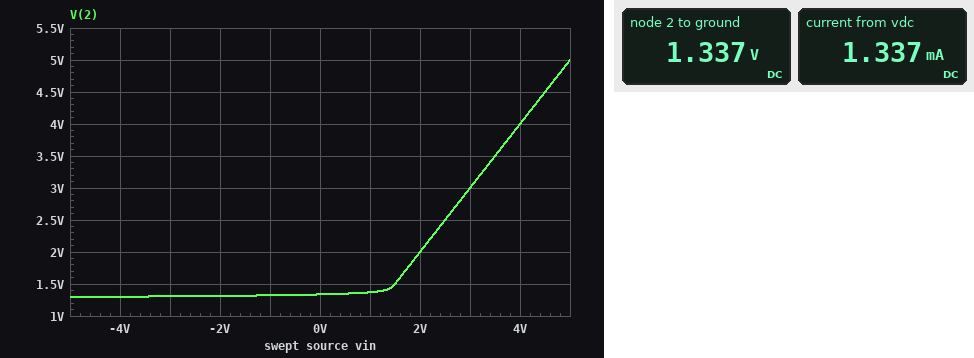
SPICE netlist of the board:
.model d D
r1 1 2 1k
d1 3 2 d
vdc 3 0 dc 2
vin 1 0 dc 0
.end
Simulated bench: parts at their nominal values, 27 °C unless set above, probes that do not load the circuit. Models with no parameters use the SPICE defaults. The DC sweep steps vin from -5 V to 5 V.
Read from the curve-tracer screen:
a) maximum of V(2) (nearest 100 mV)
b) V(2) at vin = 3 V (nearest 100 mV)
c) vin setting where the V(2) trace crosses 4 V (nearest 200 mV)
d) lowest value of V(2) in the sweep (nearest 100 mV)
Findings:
5.0 V
3.0 V
4.0 V
1.3 V
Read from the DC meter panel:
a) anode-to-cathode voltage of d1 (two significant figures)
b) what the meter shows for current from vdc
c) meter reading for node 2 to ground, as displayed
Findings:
660 mV
1.337 mA
1.337 V
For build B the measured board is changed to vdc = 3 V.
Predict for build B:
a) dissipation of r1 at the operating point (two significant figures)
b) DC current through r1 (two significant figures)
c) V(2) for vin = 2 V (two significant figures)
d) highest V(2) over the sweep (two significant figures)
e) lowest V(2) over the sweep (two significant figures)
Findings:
5.4 mW
2.3 mA
2.4 V
5.0 V
2.3 V
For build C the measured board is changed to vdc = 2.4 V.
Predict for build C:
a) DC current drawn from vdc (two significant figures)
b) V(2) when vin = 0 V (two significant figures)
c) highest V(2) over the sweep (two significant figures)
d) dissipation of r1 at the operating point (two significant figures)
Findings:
1.7 mA
1.7 V
5.0 V
3.0 mW
